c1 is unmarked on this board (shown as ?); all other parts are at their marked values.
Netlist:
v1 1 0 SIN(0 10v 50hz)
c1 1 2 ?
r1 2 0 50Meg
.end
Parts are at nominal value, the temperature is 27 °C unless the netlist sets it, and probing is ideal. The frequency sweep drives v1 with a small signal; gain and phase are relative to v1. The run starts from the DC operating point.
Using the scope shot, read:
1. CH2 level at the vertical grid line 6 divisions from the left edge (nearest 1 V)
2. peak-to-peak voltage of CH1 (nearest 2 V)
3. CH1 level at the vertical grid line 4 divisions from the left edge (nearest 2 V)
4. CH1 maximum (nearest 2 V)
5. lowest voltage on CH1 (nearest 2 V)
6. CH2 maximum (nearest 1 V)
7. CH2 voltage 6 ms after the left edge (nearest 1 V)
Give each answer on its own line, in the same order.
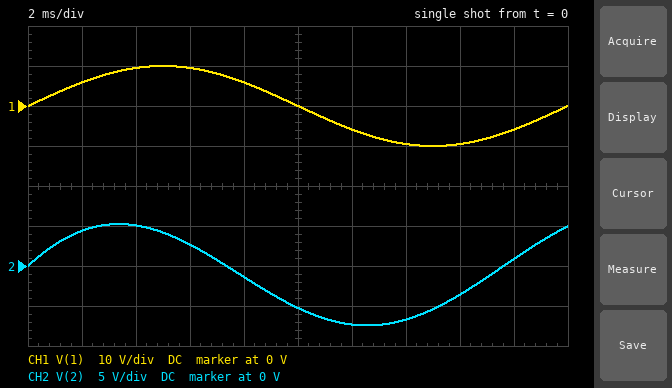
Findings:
-7 V
20 V
6 V
10 V
-10 V
5 V
3 V
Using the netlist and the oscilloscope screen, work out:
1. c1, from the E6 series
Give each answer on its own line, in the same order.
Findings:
68 pF
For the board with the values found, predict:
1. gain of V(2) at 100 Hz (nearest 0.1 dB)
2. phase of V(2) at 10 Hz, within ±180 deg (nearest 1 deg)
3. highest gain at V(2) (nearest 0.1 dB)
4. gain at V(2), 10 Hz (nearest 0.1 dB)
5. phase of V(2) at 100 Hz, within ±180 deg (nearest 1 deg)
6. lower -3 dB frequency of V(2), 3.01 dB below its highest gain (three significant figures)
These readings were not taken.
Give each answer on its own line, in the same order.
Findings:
-0.9 dB
78 deg
0 dB
-13.6 dB
25 deg
46.8 Hz
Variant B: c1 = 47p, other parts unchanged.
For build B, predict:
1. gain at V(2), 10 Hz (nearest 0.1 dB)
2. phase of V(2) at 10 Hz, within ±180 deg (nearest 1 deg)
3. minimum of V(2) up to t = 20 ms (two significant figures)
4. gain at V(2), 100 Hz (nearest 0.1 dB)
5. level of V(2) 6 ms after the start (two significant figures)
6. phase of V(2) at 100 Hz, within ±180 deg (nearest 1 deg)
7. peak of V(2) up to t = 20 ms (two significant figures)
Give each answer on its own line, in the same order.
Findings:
-16.7 dB
82 deg
-6.0 V
-1.6 dB
1.5 V
34 deg
4.8 V
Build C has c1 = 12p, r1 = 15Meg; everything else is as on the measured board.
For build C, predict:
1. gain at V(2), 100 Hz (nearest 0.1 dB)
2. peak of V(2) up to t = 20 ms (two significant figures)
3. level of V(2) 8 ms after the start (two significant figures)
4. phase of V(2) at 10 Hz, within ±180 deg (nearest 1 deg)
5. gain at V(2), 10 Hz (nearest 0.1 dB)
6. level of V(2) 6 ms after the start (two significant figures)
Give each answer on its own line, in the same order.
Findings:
-19.0 dB
560 mV
-440 mV
89 deg
-38.9 dB
-140 mV
